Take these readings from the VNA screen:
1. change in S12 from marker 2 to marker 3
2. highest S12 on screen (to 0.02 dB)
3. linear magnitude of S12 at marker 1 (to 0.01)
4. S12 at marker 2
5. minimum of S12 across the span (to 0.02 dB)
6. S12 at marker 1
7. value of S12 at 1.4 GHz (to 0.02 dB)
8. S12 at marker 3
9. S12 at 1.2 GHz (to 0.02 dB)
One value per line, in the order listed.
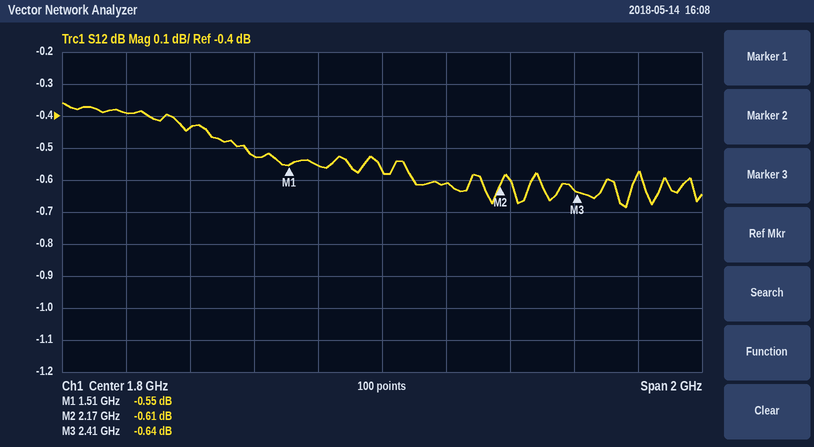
-0.03 dB
-0.36 dB
0.94
-0.61 dB
-0.68 dB
-0.55 dB
-0.52 dB
-0.64 dB
-0.44 dB
